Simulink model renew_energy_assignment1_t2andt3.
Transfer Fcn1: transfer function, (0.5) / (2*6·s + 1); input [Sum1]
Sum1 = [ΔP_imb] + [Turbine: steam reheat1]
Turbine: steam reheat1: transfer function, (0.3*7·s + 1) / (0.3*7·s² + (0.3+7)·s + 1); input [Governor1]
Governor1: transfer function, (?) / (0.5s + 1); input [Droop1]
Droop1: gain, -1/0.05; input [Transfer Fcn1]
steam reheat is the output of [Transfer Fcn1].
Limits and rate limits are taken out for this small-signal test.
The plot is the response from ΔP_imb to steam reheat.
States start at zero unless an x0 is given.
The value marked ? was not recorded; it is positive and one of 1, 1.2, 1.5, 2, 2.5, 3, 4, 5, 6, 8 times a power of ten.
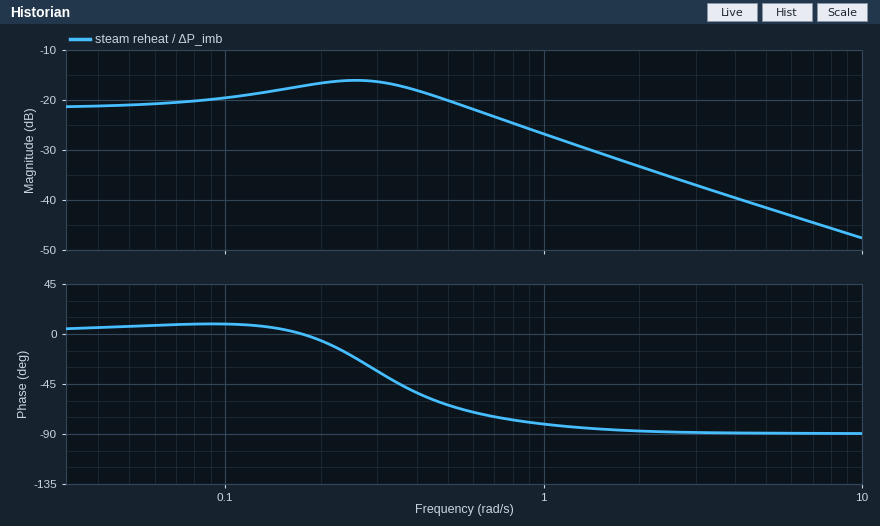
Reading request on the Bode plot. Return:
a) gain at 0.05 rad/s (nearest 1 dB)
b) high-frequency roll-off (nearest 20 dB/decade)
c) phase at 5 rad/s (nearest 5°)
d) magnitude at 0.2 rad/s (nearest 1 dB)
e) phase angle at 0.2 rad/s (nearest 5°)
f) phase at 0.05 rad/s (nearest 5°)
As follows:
-21 dB
-20 dB/decade
-90°
-17 dB
-5°
5°
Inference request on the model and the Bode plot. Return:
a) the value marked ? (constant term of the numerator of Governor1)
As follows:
0.5
